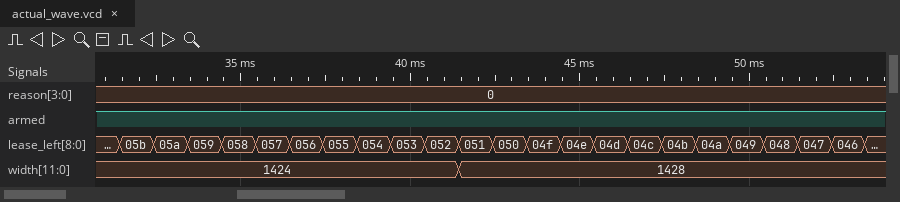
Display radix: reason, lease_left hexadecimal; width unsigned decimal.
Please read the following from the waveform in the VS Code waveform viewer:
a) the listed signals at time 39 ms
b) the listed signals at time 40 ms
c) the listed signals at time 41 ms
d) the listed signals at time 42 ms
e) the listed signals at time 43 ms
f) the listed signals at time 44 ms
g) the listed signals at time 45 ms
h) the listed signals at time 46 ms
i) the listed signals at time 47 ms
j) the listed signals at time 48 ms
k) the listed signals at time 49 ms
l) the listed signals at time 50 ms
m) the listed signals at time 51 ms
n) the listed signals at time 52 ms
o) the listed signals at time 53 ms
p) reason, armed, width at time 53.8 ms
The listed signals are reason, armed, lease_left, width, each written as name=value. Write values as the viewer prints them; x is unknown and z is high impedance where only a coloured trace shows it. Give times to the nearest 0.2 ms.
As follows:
reason=0, armed=1, lease_left=054, width=1424
reason=0, armed=1, lease_left=053, width=1424
reason=0, armed=1, lease_left=052, width=1424
reason=0, armed=1, lease_left=051, width=1428
reason=0, armed=1, lease_left=050, width=1428
reason=0, armed=1, lease_left=04f, width=1428
reason=0, armed=1, lease_left=04e, width=1428
reason=0, armed=1, lease_left=04d, width=1428
reason=0, armed=1, lease_left=04c, width=1428
reason=0, armed=1, lease_left=04b, width=1428
reason=0, armed=1, lease_left=04a, width=1428
reason=0, armed=1, lease_left=049, width=1428
reason=0, armed=1, lease_left=048, width=1428
reason=0, armed=1, lease_left=047, width=1428
reason=0, armed=1, lease_left=046, width=1428
reason=0, armed=1, width=1428
